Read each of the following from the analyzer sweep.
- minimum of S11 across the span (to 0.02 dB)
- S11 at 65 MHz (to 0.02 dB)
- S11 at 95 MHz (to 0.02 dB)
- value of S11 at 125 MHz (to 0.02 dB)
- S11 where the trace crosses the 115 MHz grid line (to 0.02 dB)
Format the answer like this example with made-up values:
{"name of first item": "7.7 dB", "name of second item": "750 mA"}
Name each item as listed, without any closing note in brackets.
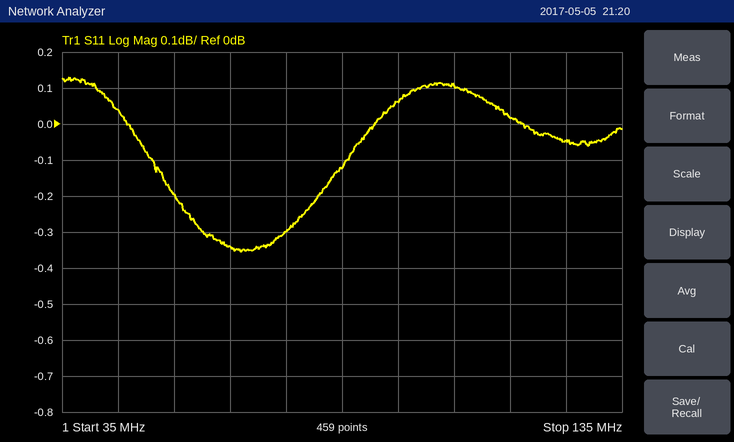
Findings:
{"minimum of S11 across the span": "-0.36 dB", "S11 at 65 MHz": "-0.34 dB", "S11 at 95 MHz": "0.06 dB", "value of S11 at 125 MHz": "-0.04 dB", "S11 where the trace crosses the 115 MHz grid line": "0.02 dB"}
